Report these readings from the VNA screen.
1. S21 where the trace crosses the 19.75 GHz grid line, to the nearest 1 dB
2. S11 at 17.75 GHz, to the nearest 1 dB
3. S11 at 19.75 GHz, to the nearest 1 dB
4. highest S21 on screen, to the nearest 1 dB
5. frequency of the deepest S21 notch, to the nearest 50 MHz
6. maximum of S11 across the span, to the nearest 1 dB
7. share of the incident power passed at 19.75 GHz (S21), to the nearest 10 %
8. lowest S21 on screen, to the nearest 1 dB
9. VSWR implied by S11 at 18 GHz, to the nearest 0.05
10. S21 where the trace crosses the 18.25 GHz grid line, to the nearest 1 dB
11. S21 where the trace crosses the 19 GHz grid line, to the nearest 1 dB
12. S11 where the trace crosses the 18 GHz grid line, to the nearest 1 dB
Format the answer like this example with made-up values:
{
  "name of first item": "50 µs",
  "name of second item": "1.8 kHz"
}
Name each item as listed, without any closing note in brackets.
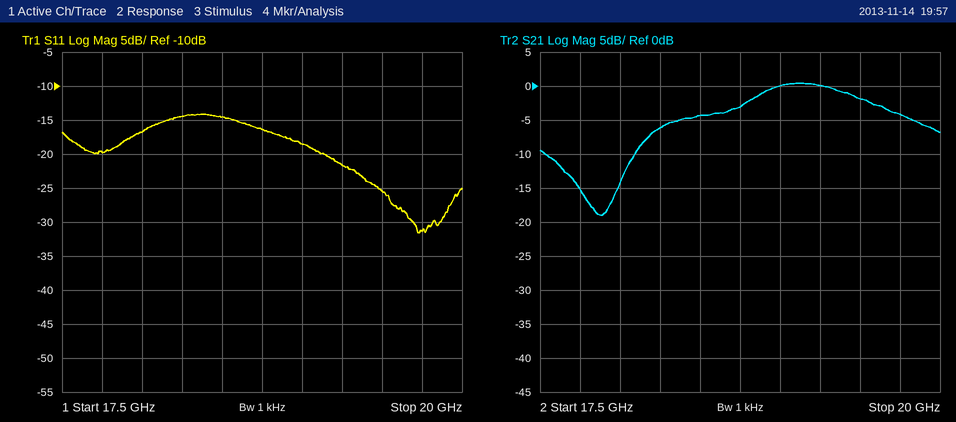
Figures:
{
  "S21 where the trace crosses the 19.75 GHz grid line, to the nearest 1 dB": "-4 dB",
  "S11 at 17.75 GHz, to the nearest 1 dB": "-20 dB",
  "S11 at 19.75 GHz, to the nearest 1 dB": "-31 dB",
  "highest S21 on screen, to the nearest 1 dB": "0 dB",
  "frequency of the deepest S21 notch, to the nearest 50 MHz": "17.90 GHz",
  "maximum of S11 across the span, to the nearest 1 dB": "-14 dB",
  "share of the incident power passed at 19.75 GHz (S21), to the nearest 10 %": "40 %",
  "lowest S21 on screen, to the nearest 1 dB": "-19 dB",
  "VSWR implied by S11 at 18 GHz, to the nearest 0.05": "1.35",
  "S21 where the trace crosses the 18.25 GHz grid line, to the nearest 1 dB": "-6 dB",
  "S21 where the trace crosses the 19 GHz grid line, to the nearest 1 dB": "0 dB",
  "S11 where the trace crosses the 18 GHz grid line, to the nearest 1 dB": "-17 dB"
}
